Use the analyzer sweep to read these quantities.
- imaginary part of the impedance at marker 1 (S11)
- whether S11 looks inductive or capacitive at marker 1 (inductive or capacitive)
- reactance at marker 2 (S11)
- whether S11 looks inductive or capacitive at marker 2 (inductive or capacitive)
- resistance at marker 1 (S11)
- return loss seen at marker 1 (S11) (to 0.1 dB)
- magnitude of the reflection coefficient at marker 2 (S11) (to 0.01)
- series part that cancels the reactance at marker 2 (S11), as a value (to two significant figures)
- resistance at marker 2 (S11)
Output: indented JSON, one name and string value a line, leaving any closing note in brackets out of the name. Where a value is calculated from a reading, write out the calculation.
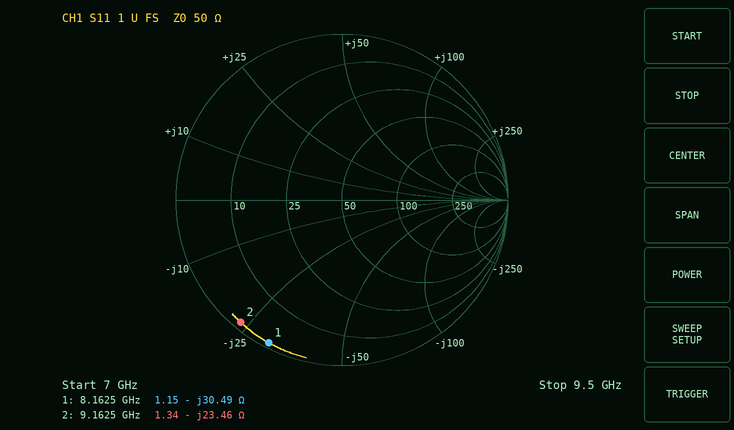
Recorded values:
{
  "imaginary part of the impedance at marker 1": "-30.49 Ω",
  "whether S11 looks inductive or capacitive at marker 1": "capacitive",
  "reactance at marker 2": "-23.46 Ω",
  "whether S11 looks inductive or capacitive at marker 2": "capacitive",
  "resistance at marker 1": "1.15 Ω",
  "return loss seen at marker 1 (S11)": "0.3 dB",
  "magnitude of the reflection coefficient at marker 2 (S11)": "0.96",
  "series part that cancels the reactance at marker 2 (S11), as a value": "L = 23.46 Ω/(2π × 9.1625 GHz) ≈ 408 pH, so 410 pH to two significant figures",
  "resistance at marker 2": "1.34 Ω"
}
